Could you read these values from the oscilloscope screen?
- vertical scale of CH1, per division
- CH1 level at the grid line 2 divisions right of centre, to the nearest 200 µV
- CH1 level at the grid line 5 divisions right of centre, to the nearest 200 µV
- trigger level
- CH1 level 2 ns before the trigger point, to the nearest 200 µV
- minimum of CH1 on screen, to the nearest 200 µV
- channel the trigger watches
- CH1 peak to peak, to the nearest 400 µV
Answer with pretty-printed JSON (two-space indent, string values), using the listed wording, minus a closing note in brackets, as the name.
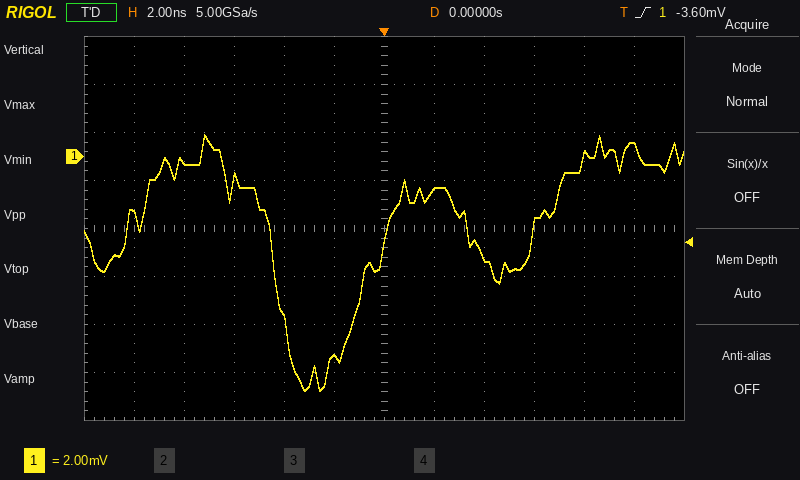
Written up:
{
  "vertical scale of CH1, per division": "2 mV",
  "CH1 level at the grid line 2 divisions right of centre, to the nearest 200 µV": "-4.2 mV",
  "CH1 level at the grid line 5 divisions right of centre, to the nearest 200 µV": "400 µV",
  "trigger level": "-3.60 mV",
  "CH1 level 2 ns before the trigger point, to the nearest 200 µV": "-8.4 mV",
  "minimum of CH1 on screen, to the nearest 200 µV": "-9.8 mV",
  "channel the trigger watches": "CH1",
  "CH1 peak to peak, to the nearest 400 µV": "10.8 mV"
}
